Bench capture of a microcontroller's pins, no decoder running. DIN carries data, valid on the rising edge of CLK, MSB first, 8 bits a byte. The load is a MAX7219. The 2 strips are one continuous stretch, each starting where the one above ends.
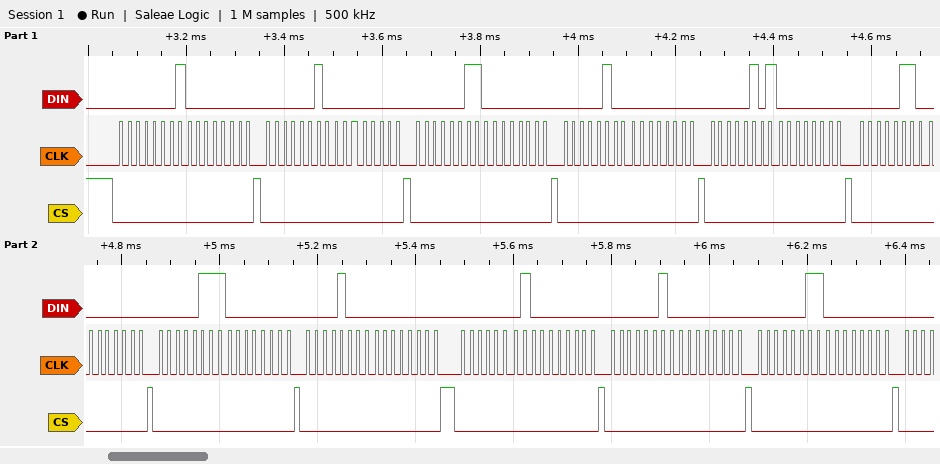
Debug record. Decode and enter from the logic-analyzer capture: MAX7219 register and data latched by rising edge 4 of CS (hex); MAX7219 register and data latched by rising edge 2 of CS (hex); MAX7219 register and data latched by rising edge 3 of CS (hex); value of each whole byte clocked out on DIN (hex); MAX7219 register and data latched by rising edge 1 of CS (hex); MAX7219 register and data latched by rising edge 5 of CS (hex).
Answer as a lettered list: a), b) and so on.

a) register 0x4, data 0x00
b) register 0x2, data 0x00
c) register 0x3, data 0x00
d) 01 00 02 00 03 00 04 00 05 00 06 00 07 00 08 00 01 00 02 00 03 00
e) register 0x1, data 0x00
f) register 0x5, data 0x00
